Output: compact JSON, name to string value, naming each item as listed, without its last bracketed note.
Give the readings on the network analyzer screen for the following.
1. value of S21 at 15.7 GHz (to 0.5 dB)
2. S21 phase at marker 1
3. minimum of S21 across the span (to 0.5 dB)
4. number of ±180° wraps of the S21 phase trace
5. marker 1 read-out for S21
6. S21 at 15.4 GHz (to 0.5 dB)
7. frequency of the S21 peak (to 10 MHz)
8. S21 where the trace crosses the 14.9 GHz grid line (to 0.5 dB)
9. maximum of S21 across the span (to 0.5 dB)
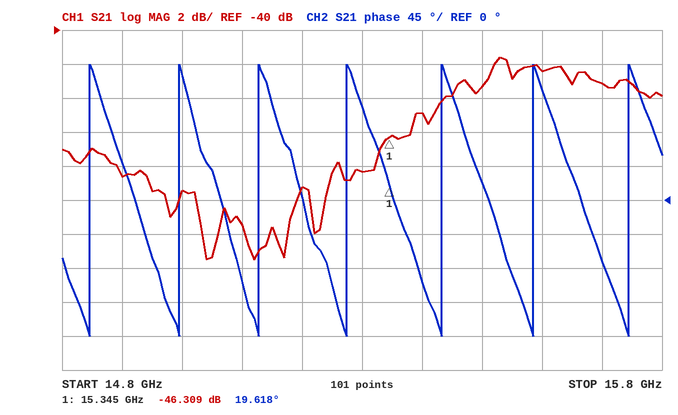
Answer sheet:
{"value of S21 at 15.7 GHz": "-43.0 dB", "S21 phase at marker 1": "19.618°", "minimum of S21 across the span": "-53.5 dB", "number of ±180° wraps of the S21 phase trace": "7", "marker 1 read-out for S21": "-46.309 dB", "S21 at 15.4 GHz": "-45.0 dB", "frequency of the S21 peak": "15.53 GHz", "S21 where the trace crosses the 14.9 GHz grid line": "-48.5 dB", "maximum of S21 across the span": "-41.5 dB"}
